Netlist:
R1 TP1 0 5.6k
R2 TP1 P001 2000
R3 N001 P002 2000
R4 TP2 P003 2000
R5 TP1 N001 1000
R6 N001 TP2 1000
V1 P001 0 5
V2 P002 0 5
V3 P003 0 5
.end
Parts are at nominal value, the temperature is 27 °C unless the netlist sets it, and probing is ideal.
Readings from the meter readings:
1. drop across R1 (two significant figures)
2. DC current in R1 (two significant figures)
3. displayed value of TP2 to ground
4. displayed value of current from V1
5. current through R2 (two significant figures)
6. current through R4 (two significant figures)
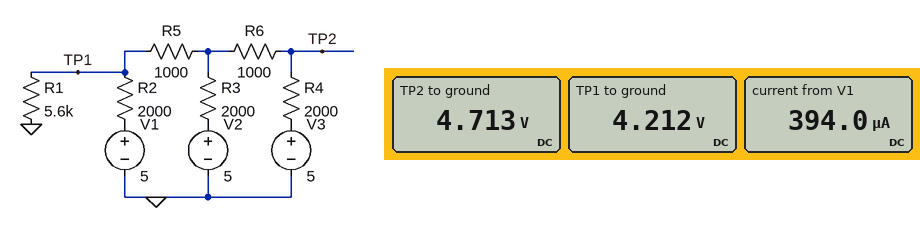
4.2 V
750 µA
4.713 V
394.0 µA
390 µA
140 µA
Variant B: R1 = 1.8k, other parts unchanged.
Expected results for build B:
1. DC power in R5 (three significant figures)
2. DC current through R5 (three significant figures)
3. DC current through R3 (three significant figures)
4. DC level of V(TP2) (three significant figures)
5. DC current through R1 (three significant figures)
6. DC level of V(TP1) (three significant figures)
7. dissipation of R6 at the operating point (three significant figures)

699 µW
836 µA
502 µA
4.33 V
1.76 mA
3.16 V
112 µW
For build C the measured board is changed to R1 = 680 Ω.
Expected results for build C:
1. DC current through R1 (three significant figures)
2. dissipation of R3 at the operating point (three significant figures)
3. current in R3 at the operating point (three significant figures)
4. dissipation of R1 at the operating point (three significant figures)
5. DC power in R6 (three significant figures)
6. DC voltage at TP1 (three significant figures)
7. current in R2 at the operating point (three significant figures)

2.89 mA
1.37 mW
827 µA
5.70 mW
304 µW
1.97 V
1.52 mA
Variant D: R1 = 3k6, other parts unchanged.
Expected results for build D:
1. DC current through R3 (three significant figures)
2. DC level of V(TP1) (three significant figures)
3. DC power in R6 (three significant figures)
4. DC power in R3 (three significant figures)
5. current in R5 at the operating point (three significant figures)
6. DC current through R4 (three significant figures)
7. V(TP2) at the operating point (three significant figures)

307 µA
3.87 V
42.0 µW
189 µW
512 µA
205 µA
4.59 V
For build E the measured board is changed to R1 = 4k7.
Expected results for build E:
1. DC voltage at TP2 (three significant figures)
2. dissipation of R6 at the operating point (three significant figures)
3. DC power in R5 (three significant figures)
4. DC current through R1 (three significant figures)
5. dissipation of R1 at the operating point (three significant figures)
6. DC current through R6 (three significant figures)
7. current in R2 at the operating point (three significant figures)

4.67 V
27.5 µW
172 µW
870 µA
3.56 mW
166 µA
456 µA
